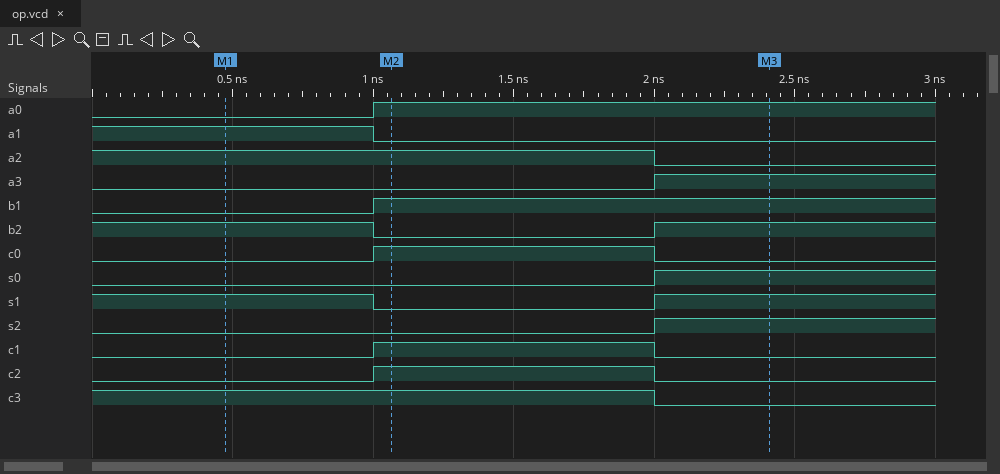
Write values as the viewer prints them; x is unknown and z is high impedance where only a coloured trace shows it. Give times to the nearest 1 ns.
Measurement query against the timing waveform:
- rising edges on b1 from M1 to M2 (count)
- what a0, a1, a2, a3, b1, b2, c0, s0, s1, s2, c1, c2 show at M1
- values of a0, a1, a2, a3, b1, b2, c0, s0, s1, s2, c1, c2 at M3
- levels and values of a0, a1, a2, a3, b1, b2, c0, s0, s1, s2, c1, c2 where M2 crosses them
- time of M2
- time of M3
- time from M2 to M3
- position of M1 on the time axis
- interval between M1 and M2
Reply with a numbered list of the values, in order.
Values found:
1. 1
2. a0=0, a1=1, a2=1, a3=0, b1=0, b2=1, c0=0, s0=0, s1=1, s2=0, c1=0, c2=0
3. a0=1, a1=0, a2=0, a3=1, b1=1, b2=1, c0=0, s0=1, s1=1, s2=1, c1=0, c2=0
4. a0=1, a1=0, a2=1, a3=0, b1=1, b2=0, c0=1, s0=0, s1=0, s2=0, c1=1, c2=1
5. 1 ns
6. 2 ns
7. 1 ns
8. 0 ns
9. 1 ns
